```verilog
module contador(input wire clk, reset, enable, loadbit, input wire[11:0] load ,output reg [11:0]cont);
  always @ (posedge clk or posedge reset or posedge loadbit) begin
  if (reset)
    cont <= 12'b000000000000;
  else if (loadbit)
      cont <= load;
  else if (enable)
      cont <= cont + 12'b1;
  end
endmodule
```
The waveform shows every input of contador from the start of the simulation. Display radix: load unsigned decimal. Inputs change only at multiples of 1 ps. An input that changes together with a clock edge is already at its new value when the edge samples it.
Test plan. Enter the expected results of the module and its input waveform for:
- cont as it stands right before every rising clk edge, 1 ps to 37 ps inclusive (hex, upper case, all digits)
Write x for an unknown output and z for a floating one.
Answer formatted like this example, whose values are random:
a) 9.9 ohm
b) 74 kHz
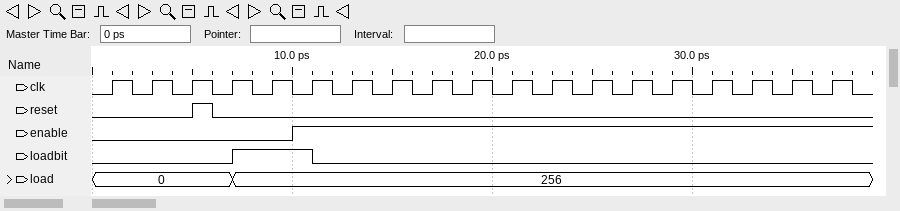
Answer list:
a) x, x, x, 000, 100, 100, 101, 102, 103, 104, 105, 106, 107, 108, 109, 10A, 10B, 10C, 10D
